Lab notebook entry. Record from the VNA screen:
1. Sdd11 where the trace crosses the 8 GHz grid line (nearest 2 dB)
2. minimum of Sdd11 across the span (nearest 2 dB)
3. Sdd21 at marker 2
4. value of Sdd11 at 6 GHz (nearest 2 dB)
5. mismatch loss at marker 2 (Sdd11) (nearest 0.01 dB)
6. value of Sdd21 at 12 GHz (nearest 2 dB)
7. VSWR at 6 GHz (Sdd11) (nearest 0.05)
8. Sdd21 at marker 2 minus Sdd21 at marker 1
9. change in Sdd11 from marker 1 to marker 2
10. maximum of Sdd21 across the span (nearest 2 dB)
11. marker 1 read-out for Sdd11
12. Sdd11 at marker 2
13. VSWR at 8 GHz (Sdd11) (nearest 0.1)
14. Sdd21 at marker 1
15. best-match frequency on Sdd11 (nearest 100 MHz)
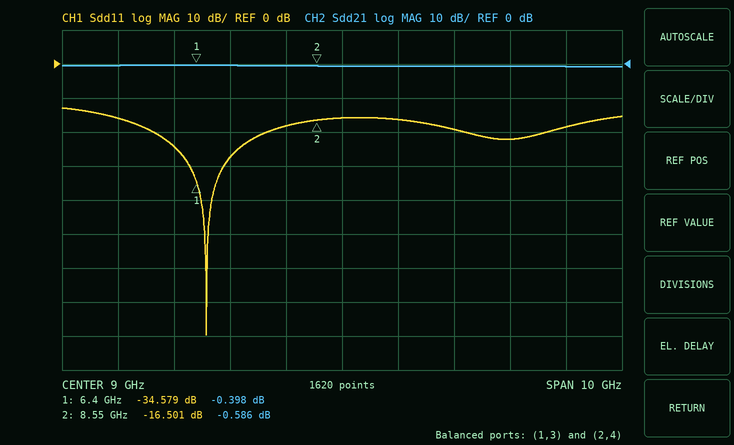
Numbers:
-18 dB
-80 dB
-0.586 dB
-24 dB
0.10 dB
0 dB
1.15
-0.188 dB
18.078 dB
0 dB
-34.579 dB
-16.501 dB
1.3
-0.398 dB
6.6 GHz
